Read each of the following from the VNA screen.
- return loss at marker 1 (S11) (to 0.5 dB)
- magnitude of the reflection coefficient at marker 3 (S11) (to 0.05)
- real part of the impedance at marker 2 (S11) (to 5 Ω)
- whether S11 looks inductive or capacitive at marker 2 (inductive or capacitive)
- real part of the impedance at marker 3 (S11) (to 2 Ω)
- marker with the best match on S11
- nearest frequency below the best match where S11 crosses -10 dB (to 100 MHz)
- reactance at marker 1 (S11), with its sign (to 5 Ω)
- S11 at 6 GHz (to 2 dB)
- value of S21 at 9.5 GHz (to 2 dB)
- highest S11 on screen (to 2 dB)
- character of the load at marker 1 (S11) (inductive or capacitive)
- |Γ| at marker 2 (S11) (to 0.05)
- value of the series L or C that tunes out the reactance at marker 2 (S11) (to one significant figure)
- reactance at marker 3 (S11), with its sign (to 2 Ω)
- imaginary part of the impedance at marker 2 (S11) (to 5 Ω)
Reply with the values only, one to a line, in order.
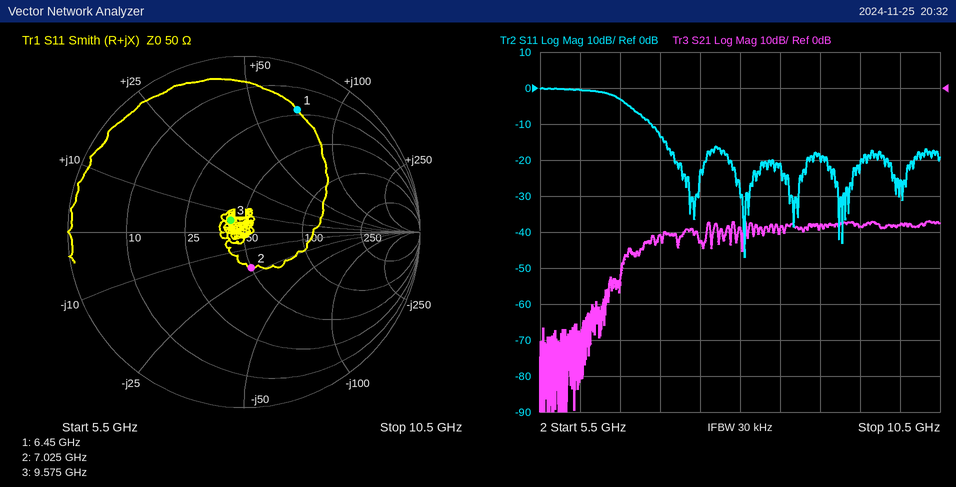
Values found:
2.5 dB
0.10
50 Ω
capacitive
42 Ω
marker 3
6.9 GHz
+70 Ω
0 dB
-38 dB
0 dB
inductive
0.20
500 pH
+6 Ω
-20 Ω
